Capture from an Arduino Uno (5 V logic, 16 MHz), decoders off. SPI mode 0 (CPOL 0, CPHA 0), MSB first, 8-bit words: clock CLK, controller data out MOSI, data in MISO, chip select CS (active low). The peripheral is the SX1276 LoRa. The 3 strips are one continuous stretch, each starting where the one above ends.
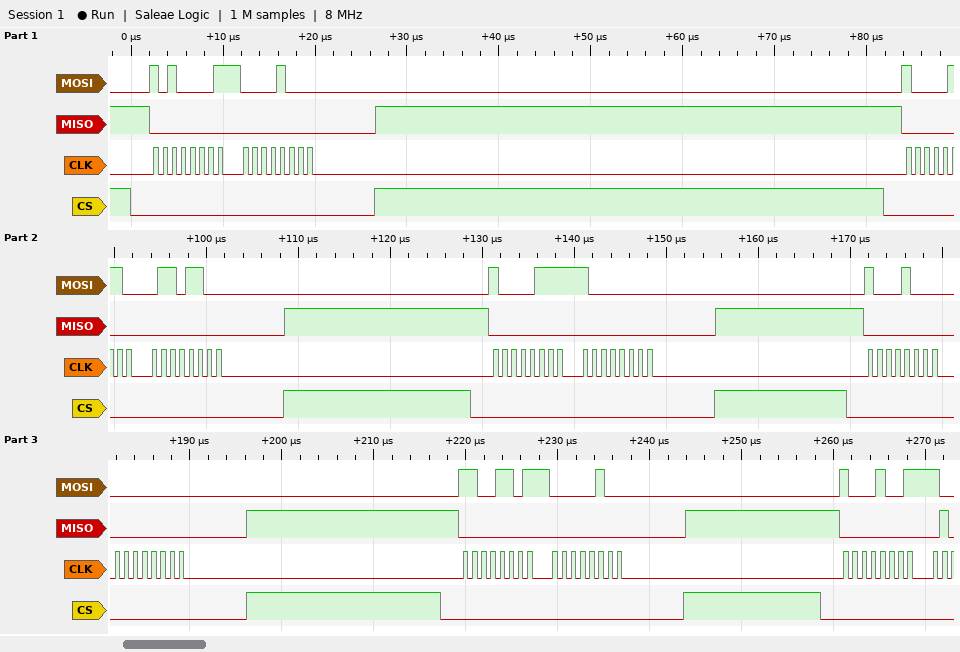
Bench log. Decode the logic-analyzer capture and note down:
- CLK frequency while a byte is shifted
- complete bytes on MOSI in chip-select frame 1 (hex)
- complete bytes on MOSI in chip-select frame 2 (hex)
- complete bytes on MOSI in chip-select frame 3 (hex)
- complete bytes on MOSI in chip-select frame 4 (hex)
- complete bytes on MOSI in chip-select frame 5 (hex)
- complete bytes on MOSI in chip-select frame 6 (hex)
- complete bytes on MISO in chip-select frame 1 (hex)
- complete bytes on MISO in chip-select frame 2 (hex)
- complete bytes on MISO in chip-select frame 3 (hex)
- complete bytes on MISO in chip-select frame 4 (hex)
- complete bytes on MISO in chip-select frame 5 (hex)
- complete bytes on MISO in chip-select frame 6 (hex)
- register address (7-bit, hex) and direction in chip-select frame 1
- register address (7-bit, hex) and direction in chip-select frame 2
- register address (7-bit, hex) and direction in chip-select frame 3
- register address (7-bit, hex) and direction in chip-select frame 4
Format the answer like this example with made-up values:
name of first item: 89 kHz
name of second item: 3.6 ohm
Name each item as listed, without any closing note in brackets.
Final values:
CLK frequency while a byte is shifted: 1 MHz
complete bytes on MOSI in chip-select frame 1: A1 08
complete bytes on MOSI in chip-select frame 2: 86 6C
complete bytes on MOSI in chip-select frame 3: 87 80
complete bytes on MOSI in chip-select frame 4: 88 00
complete bytes on MOSI in chip-select frame 5: CD 04
complete bytes on MOSI in chip-select frame 6: 89
complete bytes on MISO in chip-select frame 1: 00 00
complete bytes on MISO in chip-select frame 2: 00 00
complete bytes on MISO in chip-select frame 3: 00 00
complete bytes on MISO in chip-select frame 4: 00 00
complete bytes on MISO in chip-select frame 5: 00 00
complete bytes on MISO in chip-select frame 6: 00
register address (7-bit, hex) and direction in chip-select frame 1: 0x21 write
register address (7-bit, hex) and direction in chip-select frame 2: 0x06 write
register address (7-bit, hex) and direction in chip-select frame 3: 0x07 write
register address (7-bit, hex) and direction in chip-select frame 4: 0x08 write
